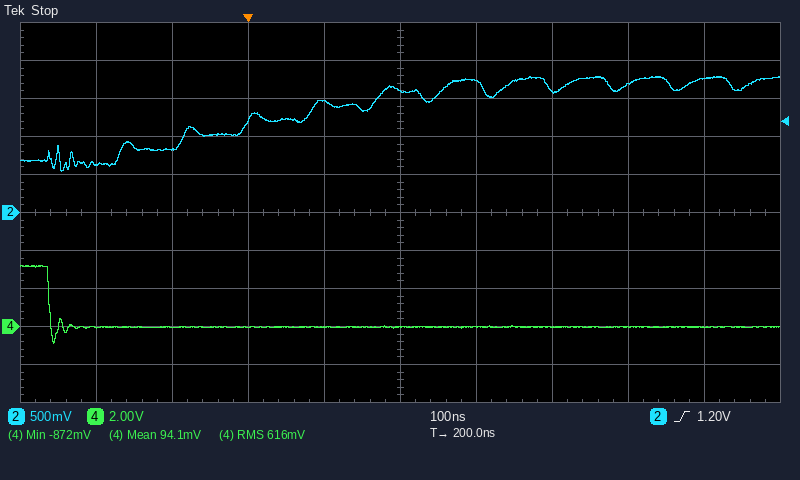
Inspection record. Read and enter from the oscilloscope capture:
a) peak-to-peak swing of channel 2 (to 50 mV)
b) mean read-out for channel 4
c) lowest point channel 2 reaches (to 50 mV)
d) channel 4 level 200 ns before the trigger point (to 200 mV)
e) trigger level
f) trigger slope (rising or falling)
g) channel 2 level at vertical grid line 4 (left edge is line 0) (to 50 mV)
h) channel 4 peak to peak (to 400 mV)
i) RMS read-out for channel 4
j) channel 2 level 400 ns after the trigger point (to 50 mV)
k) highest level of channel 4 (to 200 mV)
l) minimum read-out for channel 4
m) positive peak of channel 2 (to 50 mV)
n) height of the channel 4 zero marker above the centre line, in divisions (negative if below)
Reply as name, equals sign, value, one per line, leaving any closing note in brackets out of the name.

peak-to-peak swing of channel 2 = 1.25 V
mean read-out for channel 4 = 94.1 mV
lowest point channel 2 reaches = 550 mV
channel 4 level 200 ns before the trigger point = 0.0 V
trigger level = 1.20 V
trigger slope = rising
channel 2 level at vertical grid line 4 (left edge is line 0) = 1.45 V
channel 4 peak to peak = 4.0 V
RMS read-out for channel 4 = 616 mV
channel 2 level 400 ns after the trigger point = 1.60 V
highest level of channel 4 = 3.2 V
minimum read-out for channel 4 = -872 mV
positive peak of channel 2 = 1.80 V
height of the channel 4 zero marker above the centre line, in divisions = -3.0 div
